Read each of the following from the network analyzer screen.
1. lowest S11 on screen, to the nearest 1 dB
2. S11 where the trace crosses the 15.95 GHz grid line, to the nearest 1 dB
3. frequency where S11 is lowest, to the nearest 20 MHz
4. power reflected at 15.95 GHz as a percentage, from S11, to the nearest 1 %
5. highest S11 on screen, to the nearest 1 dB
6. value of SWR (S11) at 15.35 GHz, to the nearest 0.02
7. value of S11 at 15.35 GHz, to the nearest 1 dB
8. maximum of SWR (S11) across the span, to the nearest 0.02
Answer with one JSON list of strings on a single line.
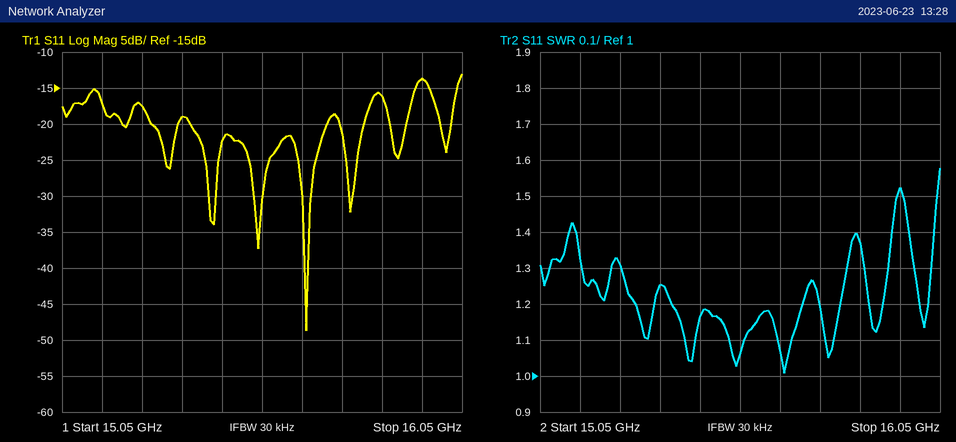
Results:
["-49 dB", "-14 dB", "15.66 GHz", "4 %", "-13 dB", "1.26", "-19 dB", "1.58"]
